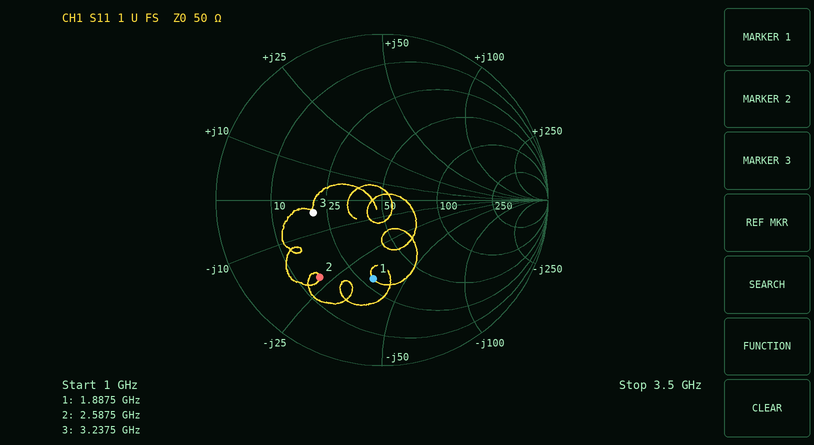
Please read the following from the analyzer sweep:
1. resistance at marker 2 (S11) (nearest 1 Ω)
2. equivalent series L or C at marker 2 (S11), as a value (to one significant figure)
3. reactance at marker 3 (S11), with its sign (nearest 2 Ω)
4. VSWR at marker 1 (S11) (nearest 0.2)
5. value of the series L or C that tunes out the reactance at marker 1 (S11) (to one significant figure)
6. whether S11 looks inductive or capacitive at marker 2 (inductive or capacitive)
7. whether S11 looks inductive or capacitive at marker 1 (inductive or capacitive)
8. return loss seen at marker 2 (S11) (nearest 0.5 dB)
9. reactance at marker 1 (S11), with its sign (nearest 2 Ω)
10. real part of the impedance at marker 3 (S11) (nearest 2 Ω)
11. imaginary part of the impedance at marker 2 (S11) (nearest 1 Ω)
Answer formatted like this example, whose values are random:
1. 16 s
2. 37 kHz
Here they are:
1. 15 Ω
2. 3 pF
3. -4 Ω
4. 2.8
5. 3 nH
6. capacitive
7. capacitive
8. 4.5 dB
9. -36 Ω
10. 20 Ω
11. -22 Ω
